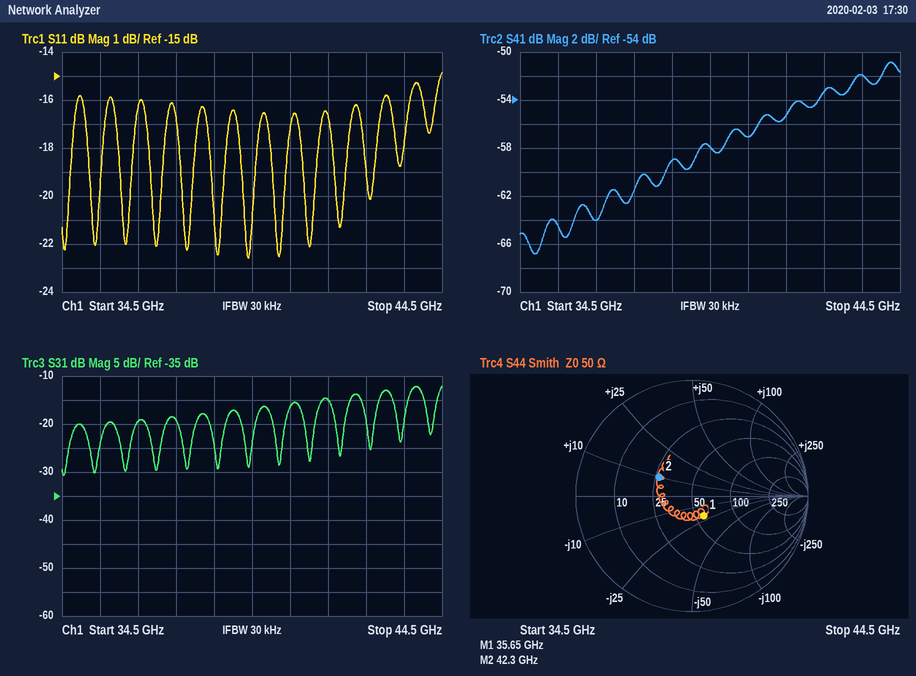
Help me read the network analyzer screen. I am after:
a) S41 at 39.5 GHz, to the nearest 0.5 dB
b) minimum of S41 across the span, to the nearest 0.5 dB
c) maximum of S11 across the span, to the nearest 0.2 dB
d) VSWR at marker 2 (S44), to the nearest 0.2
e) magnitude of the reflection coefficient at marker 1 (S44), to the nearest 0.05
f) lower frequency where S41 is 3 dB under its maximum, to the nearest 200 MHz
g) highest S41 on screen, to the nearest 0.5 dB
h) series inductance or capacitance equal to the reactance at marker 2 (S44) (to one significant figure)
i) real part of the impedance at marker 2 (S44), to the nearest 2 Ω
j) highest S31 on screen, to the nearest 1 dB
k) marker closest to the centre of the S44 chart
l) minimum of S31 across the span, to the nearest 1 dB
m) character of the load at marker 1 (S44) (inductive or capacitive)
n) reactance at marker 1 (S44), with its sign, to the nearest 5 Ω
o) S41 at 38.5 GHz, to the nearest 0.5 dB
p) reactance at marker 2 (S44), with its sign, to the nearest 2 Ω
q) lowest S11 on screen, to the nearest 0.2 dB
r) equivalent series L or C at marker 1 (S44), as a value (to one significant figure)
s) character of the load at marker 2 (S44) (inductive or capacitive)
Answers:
-58.0 dB
-67.0 dB
-14.8 dB
2.0
0.20
42.4 GHz
-51.0 dB
40 pH
26 Ω
-12 dB
marker 1
-31 dB
capacitive
-20 Ω
-59.0 dB
+10 Ω
-22.6 dB
200 fF
inductive
